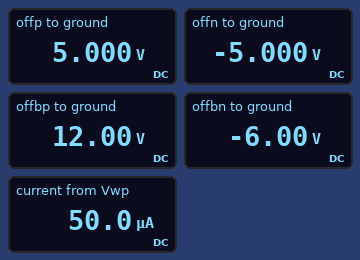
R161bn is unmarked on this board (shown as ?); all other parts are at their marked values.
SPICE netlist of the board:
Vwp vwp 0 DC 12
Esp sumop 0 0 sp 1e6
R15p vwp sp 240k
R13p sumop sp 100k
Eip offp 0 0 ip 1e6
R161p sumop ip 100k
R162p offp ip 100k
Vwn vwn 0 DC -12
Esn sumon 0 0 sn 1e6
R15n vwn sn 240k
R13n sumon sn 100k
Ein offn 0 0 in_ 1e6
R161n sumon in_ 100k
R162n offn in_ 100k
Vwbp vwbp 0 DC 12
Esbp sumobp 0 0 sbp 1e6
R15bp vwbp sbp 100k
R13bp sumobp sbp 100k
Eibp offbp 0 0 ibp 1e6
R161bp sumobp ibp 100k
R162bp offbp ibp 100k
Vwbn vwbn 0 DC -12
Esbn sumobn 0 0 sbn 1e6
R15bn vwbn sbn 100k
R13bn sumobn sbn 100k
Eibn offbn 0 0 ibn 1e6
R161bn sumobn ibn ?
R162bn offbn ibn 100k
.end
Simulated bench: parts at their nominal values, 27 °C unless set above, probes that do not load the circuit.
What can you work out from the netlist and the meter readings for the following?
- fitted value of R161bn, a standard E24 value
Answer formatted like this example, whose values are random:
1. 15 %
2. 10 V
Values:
1. 200 kΩ
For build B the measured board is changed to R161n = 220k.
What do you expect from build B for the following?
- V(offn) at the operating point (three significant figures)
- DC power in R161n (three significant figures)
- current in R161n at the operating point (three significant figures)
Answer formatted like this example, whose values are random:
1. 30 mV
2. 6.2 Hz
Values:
1. -2.27 V
2. 114 µW
3. 22.7 µA
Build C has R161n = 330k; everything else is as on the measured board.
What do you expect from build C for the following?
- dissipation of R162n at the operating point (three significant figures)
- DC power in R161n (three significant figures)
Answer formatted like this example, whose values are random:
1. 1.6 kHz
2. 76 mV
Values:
1. 23.0 µW
2. 75.8 µW
